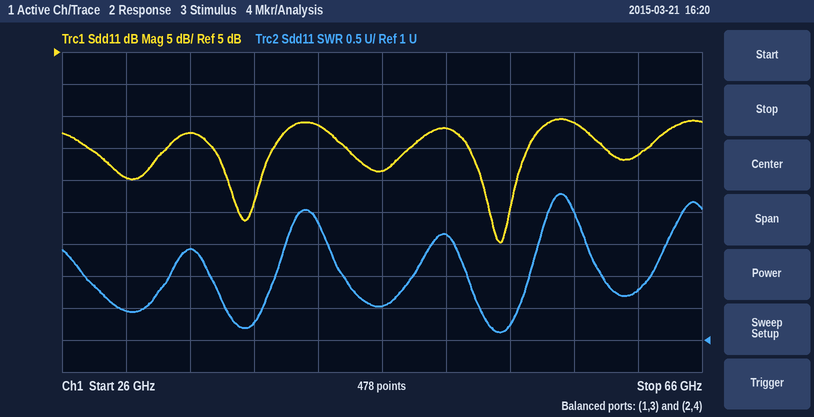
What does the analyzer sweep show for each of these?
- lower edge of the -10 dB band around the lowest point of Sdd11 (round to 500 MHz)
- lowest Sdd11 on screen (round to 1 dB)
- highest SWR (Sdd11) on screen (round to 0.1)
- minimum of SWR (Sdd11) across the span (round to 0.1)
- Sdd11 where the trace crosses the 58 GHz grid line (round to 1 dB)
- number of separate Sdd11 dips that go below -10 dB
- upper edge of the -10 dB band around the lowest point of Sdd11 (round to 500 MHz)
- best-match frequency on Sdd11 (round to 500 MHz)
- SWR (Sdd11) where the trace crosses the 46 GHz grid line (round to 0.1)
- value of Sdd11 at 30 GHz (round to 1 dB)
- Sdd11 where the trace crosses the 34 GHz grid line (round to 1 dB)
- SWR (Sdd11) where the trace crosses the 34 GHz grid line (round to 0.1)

51.5 GHz
-25 dB
3.3
1.1
-6 dB
5
55.0 GHz
53.5 GHz
1.5
-15 dB
-8 dB
2.4
